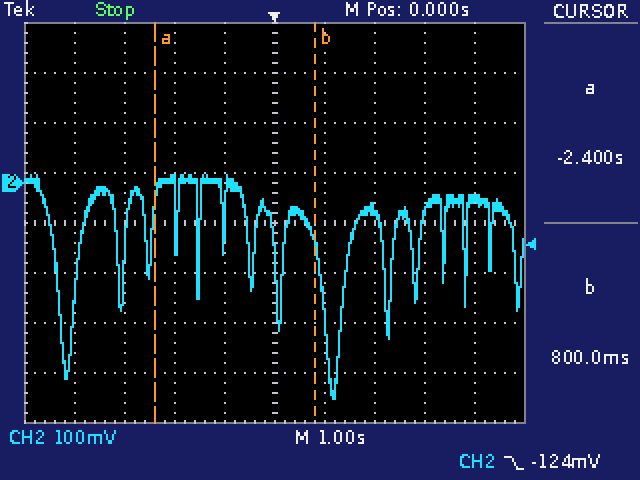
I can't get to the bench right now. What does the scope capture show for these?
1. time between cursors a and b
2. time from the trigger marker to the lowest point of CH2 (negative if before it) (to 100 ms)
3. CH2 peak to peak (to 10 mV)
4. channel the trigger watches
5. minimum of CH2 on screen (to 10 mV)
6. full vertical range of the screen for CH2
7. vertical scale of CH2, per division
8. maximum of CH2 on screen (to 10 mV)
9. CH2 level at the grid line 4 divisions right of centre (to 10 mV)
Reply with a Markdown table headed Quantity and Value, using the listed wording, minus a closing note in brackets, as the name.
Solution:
| Quantity | Value |
|---|---|
| time between cursors a and b | 3.2 s |
| time from the trigger marker to the lowest point of CH2 (negative if before it) | +1.2 s |
| CH2 peak to peak | 450 mV |
| channel the trigger watches | CH2 |
| minimum of CH2 on screen | -430 mV |
| full vertical range of the screen for CH2 | 800 mV |
| vertical scale of CH2, per division | 100 mV |
| maximum of CH2 on screen | 20 mV |
| CH2 level at the grid line 4 divisions right of centre | -30 mV |
